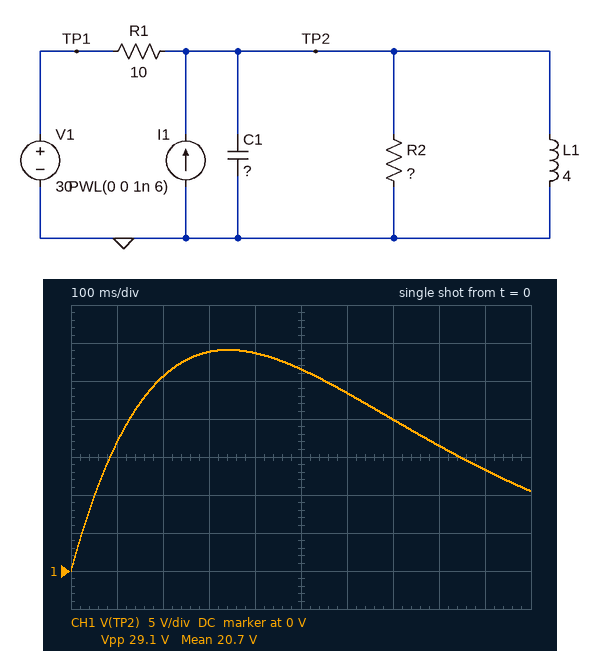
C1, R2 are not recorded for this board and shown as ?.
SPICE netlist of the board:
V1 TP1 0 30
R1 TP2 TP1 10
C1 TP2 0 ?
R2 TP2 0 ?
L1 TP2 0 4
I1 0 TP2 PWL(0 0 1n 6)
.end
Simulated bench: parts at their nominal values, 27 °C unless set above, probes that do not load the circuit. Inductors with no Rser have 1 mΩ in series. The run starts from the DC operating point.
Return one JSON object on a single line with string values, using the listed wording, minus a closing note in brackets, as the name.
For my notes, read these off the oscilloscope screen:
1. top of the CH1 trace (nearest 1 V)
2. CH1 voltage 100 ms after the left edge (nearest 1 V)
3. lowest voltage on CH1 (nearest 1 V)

{"top of the CH1 trace": "29 V", "CH1 voltage 100 ms after the left edge": "17 V", "lowest voltage on CH1": "0 V"}
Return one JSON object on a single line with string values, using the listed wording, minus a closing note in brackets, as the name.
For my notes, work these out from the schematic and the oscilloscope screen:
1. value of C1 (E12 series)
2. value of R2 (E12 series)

{"value of C1": "27 mF", "value of R2": "22 Ω"}
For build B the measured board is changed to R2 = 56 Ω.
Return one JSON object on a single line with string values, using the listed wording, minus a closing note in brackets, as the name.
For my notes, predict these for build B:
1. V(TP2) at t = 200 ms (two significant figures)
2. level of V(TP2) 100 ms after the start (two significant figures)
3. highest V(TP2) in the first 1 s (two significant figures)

{"V(TP2) at t = 200 ms": "28 V", "level of V(TP2) 100 ms after the start": "18 V", "highest V(TP2) in the first 1 s": "33 V"}
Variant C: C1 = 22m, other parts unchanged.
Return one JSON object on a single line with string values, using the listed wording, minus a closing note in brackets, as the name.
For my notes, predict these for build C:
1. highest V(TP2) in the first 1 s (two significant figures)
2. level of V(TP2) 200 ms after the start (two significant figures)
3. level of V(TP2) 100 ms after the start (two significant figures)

{"highest V(TP2) in the first 1 s": "30 V", "level of V(TP2) 200 ms after the start": "28 V", "level of V(TP2) 100 ms after the start": "20 V"}
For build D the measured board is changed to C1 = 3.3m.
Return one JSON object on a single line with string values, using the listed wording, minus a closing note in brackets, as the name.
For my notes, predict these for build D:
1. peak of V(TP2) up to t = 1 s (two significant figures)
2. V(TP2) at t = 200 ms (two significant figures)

{"peak of V(TP2) up to t = 1 s": "37 V", "V(TP2) at t = 200 ms": "31 V"}
